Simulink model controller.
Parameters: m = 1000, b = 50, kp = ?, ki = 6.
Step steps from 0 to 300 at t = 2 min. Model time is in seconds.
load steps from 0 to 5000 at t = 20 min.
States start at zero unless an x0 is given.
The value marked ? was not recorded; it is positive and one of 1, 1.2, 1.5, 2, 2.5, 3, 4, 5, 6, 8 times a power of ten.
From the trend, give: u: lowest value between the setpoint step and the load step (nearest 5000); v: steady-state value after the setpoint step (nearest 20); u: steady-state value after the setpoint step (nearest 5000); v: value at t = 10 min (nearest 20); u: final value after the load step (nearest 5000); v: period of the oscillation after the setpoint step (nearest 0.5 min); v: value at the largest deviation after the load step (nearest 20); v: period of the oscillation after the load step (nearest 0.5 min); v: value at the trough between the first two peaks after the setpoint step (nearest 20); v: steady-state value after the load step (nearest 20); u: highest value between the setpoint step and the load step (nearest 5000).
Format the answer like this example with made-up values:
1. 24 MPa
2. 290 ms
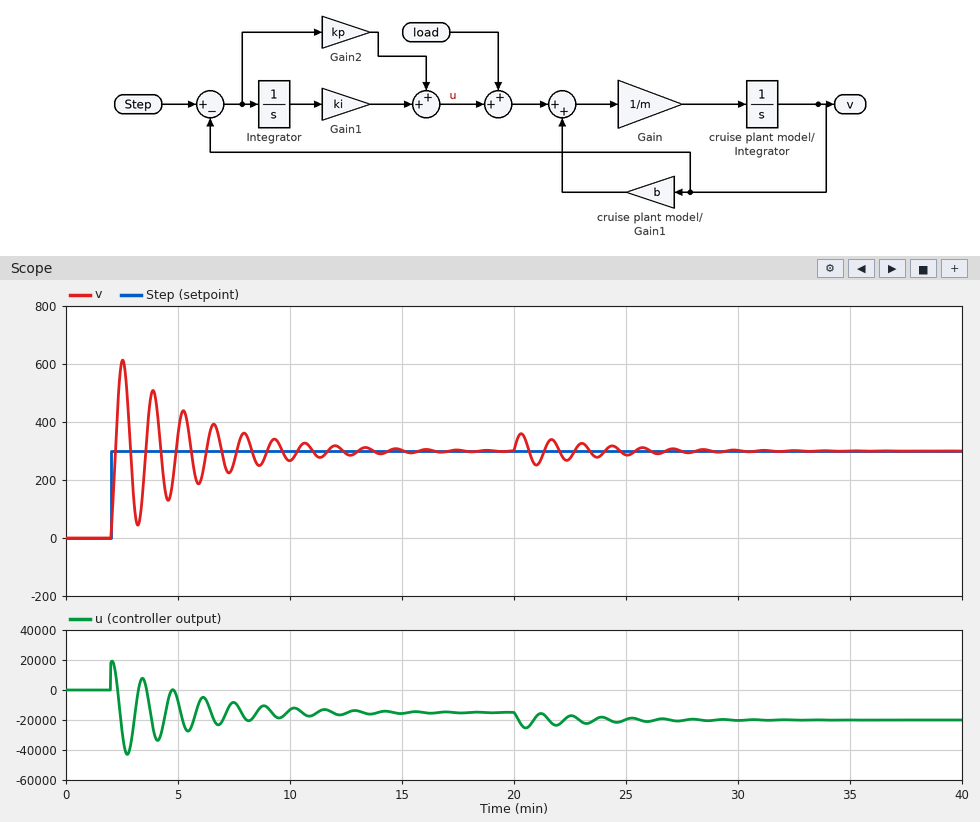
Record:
1. -45000
2. 300
3. -15000
4. 260
5. -20000
6. 1.5 min
7. 360
8. 1.5 min
9. 40
10. 300
11. 20000
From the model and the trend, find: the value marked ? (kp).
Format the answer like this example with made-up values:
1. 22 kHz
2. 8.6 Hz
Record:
1. 60
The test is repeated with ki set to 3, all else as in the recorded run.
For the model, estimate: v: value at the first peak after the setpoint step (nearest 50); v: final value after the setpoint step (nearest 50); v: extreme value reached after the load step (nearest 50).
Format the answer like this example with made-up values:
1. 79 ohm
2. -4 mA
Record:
1. 650
2. 300
3. 400
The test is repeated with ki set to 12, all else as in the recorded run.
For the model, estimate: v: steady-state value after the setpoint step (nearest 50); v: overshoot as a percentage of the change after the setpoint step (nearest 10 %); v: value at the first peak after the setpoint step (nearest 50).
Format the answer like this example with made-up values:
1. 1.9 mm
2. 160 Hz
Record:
1. 300
2. 100 %
3. 600
